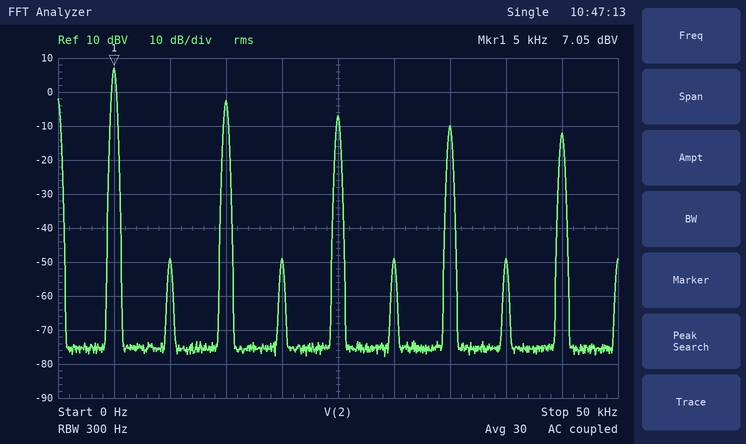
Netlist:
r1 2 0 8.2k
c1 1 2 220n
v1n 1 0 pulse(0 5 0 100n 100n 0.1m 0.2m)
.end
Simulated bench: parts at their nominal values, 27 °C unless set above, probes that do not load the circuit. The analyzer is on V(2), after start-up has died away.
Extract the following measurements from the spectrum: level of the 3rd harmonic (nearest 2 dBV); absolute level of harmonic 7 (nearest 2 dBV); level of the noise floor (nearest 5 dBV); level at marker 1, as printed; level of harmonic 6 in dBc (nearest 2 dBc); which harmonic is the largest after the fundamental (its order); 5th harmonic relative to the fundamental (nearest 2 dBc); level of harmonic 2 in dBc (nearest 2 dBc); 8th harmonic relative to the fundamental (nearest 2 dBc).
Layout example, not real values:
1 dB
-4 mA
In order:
-2 dBV
-10 dBV
-75 dBV
7.05 dBV
-56 dBc
3
-14 dBc
-56 dBc
-56 dBc
